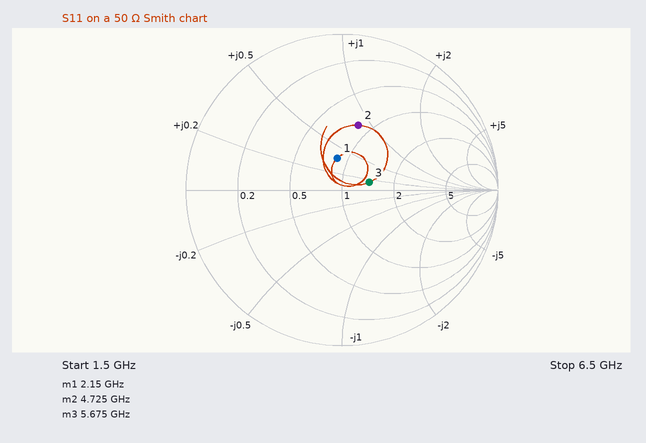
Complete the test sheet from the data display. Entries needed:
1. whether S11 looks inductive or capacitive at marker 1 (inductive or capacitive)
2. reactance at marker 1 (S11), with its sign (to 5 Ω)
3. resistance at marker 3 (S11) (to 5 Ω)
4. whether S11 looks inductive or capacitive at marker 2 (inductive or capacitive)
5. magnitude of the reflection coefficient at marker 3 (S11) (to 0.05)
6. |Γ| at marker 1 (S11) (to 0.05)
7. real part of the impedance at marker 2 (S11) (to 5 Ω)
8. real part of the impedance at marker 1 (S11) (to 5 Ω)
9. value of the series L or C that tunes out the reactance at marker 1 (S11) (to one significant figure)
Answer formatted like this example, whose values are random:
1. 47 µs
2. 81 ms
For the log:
1. inductive
2. +20 Ω
3. 70 Ω
4. inductive
5. 0.20
6. 0.20
7. 40 Ω
8. 45 Ω
9. 4 pF
